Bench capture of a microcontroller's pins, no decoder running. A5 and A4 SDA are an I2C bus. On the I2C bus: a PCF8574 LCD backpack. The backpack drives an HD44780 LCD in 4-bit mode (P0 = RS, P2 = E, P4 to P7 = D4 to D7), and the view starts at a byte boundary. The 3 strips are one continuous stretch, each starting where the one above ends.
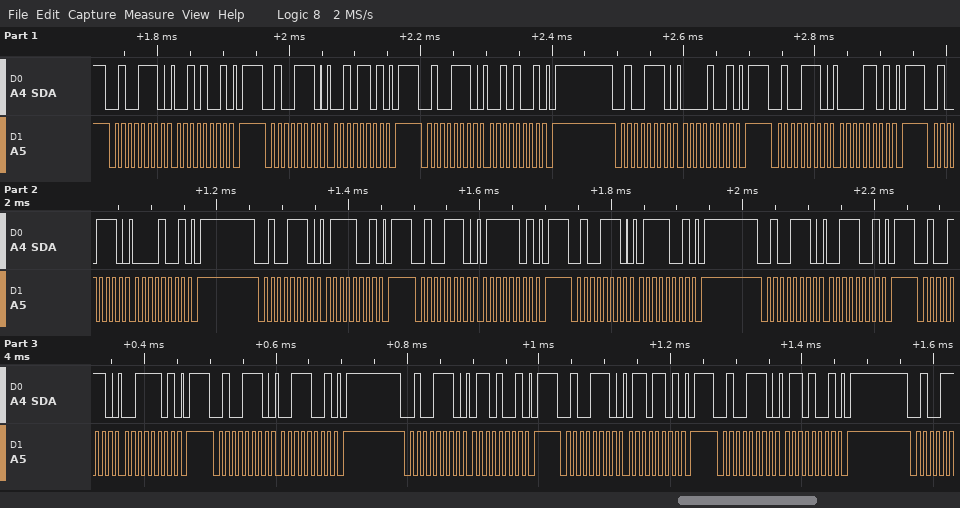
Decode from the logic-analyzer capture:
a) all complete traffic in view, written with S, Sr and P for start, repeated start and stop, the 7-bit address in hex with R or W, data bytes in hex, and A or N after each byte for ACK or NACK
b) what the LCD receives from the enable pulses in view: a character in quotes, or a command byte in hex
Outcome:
S 27W A 29 A P S 27W A 2D A P S 27W A 29 A P S 27W A 09 A P S 27W A 0D A P S 27W A 09 A P S 27W A 79 A P S 27W A 7D A P S 27W A 79 A P S 27W A 39 A P S 27W A 3D A P S 27W A 39 A P S 27W A 69 A P S 27W A 6D A P S 27W A 69 A P
' ' 's'
